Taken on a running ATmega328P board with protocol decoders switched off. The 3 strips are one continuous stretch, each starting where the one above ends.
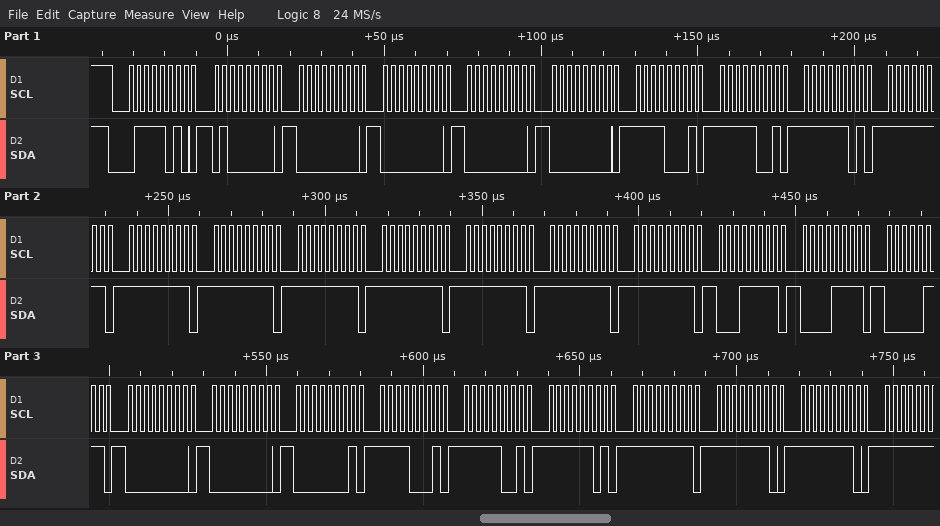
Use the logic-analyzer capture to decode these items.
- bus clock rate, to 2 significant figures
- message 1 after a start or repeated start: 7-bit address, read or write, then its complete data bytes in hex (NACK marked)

400 kHz
0x3D write: 40 00 00 00 00 F1 F9 FD FF FF FF FF FF FF FF FF 1F 0F 07 00 00 01 F1 F9 FD FF FE FE
